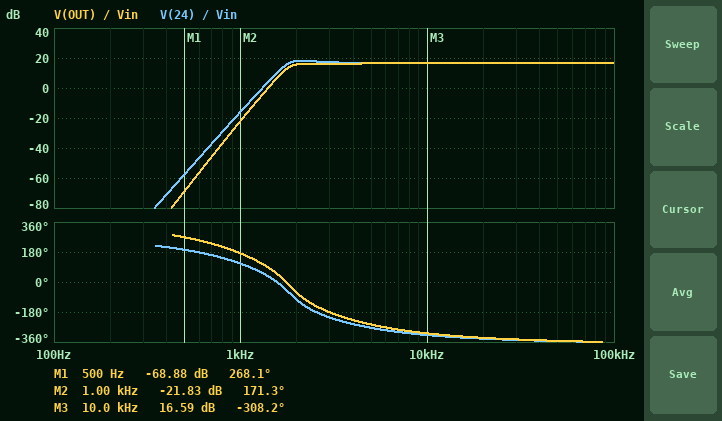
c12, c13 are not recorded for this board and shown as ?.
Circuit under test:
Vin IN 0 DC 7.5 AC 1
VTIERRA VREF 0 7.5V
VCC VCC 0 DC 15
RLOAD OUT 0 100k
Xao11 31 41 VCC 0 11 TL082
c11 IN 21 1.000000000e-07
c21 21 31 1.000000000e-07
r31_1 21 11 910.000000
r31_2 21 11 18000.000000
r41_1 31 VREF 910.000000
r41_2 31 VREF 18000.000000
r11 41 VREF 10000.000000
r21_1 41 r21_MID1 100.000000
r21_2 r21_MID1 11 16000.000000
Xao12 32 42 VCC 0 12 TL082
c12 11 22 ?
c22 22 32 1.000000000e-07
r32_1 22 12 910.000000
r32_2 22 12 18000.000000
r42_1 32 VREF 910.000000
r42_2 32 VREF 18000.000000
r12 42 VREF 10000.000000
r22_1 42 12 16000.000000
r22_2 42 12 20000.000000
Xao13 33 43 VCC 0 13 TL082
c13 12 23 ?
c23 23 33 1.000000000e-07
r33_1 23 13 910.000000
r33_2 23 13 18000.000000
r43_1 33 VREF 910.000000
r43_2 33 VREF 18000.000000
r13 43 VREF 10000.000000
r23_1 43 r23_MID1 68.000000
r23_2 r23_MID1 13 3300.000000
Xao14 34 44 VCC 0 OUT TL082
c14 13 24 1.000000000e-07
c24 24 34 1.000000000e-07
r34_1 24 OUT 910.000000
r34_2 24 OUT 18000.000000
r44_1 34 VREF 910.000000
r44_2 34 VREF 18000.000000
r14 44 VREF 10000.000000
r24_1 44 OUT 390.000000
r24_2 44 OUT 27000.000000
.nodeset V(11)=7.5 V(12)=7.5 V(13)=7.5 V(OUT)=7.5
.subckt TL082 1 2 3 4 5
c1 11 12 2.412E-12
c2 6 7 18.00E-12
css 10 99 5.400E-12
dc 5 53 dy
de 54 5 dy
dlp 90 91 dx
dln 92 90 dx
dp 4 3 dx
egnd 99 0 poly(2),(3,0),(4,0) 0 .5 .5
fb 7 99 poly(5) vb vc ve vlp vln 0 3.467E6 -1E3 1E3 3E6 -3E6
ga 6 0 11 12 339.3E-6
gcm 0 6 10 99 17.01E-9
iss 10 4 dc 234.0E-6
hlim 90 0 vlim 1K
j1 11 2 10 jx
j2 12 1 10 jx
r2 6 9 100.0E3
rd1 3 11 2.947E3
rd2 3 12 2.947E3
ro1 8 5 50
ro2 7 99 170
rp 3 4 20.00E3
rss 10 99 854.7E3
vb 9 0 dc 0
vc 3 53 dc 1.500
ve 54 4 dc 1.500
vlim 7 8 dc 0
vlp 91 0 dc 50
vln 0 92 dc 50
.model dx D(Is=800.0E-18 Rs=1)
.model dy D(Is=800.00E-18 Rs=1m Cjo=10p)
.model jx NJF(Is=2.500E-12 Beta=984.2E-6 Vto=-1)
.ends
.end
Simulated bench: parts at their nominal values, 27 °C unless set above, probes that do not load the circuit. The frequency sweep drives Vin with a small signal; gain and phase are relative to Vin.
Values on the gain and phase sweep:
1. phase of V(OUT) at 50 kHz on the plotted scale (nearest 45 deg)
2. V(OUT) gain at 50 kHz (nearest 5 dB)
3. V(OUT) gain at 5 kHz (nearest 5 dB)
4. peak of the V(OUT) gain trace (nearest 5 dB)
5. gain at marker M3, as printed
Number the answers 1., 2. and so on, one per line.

1. -360 deg
2. 15 dB
3. 15 dB
4. 15 dB
5. 16.59 dB
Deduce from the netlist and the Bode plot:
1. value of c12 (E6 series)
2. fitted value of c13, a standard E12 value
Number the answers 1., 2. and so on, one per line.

1. 150 nF
2. 120 nF
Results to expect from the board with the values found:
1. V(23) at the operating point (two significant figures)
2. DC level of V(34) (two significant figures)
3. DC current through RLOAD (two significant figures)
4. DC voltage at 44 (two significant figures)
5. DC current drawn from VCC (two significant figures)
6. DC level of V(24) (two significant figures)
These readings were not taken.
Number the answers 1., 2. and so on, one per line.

1. 7.5 V
2. 7.5 V
3. 75 µA
4. 7.5 V
5. 3.9 mA
6. 7.5 V
